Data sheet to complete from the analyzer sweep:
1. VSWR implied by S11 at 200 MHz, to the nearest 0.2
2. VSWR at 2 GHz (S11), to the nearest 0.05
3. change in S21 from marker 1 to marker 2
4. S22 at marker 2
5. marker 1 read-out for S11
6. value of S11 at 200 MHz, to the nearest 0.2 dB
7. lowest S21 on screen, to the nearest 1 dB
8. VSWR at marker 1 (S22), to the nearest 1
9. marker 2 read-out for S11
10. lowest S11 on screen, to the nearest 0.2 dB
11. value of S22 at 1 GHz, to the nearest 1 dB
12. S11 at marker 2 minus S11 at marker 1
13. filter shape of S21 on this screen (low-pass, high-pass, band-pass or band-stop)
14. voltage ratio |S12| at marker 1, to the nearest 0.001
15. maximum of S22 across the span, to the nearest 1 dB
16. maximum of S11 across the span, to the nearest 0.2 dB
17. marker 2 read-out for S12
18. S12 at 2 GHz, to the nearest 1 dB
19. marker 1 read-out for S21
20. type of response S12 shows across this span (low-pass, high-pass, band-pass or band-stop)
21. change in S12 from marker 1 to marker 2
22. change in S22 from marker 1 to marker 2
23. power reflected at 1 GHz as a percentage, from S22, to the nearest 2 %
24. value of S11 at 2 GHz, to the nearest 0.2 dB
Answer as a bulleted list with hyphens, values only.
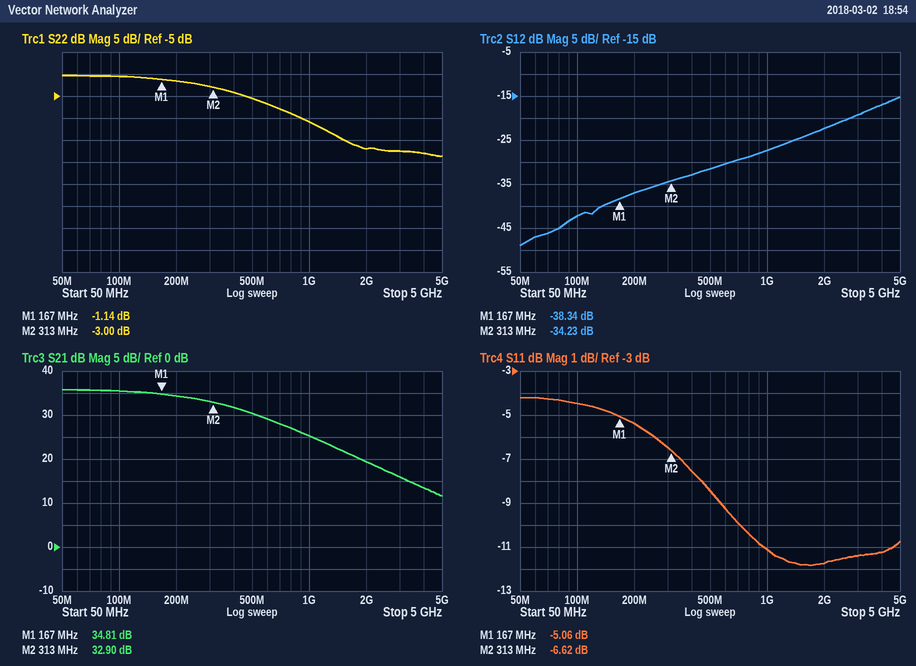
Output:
- 3.4
- 1.70
- -1.91 dB
- -3.00 dB
- -5.06 dB
- -5.4 dB
- 12 dB
- 15
- -6.62 dB
- -11.8 dB
- -11 dB
- -1.56 dB
- low-pass
- 0.012
- 0 dB
- -4.2 dB
- -34.23 dB
- -22 dB
- 34.81 dB
- high-pass
- 4.11 dB
- -1.86 dB
- 8 %
- -11.8 dB
